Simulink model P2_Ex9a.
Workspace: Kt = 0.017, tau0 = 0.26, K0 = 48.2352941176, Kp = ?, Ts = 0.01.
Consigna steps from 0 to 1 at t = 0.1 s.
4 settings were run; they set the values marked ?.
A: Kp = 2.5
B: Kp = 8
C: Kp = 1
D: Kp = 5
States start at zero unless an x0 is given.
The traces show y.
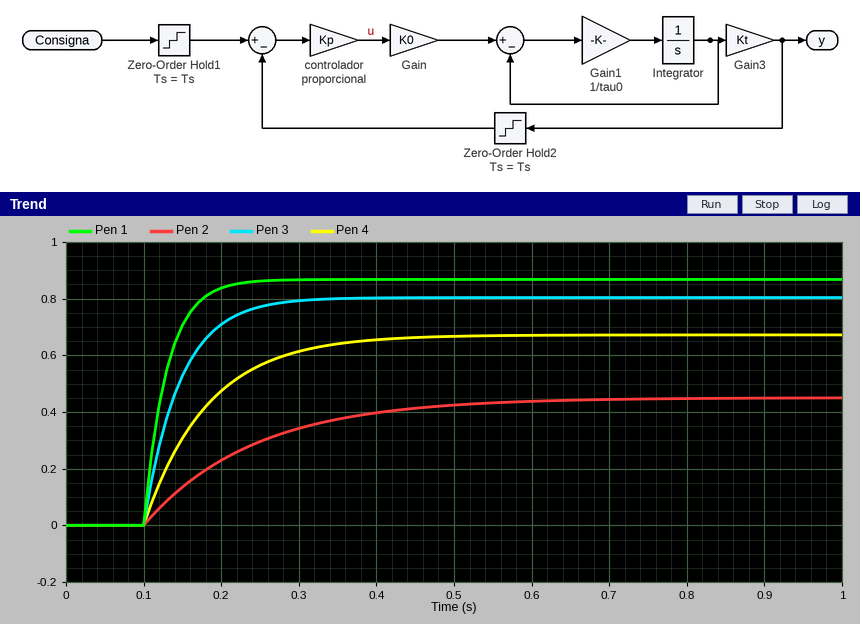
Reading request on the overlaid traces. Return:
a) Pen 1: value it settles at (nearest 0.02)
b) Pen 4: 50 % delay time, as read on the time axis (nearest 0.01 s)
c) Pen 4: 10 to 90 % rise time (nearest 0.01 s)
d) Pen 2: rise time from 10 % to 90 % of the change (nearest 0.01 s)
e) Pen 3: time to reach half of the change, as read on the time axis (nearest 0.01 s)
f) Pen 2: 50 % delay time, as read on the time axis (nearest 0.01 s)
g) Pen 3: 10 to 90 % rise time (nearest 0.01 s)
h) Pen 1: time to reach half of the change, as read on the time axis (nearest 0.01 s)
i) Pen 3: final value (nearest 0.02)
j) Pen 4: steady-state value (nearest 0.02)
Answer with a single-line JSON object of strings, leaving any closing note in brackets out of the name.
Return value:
{"Pen 1: value it settles at": "0.86", "Pen 4: 50 % delay time, as read on the time axis": "0.16 s", "Pen 4: 10 to 90 % rise time": "0.18 s", "Pen 2: rise time from 10 % to 90 % of the change": "0.31 s", "Pen 3: time to reach half of the change, as read on the time axis": "0.13 s", "Pen 2: 50 % delay time, as read on the time axis": "0.20 s", "Pen 3: 10 to 90 % rise time": "0.10 s", "Pen 1: time to reach half of the change, as read on the time axis": "0.12 s", "Pen 3: final value": "0.80", "Pen 4: steady-state value": "0.68"}
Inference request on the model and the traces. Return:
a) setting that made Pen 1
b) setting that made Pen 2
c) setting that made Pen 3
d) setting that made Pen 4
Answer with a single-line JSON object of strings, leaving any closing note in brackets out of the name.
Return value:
{"setting that made Pen 1": "B", "setting that made Pen 2": "C", "setting that made Pen 3": "D", "setting that made Pen 4": "A"}
